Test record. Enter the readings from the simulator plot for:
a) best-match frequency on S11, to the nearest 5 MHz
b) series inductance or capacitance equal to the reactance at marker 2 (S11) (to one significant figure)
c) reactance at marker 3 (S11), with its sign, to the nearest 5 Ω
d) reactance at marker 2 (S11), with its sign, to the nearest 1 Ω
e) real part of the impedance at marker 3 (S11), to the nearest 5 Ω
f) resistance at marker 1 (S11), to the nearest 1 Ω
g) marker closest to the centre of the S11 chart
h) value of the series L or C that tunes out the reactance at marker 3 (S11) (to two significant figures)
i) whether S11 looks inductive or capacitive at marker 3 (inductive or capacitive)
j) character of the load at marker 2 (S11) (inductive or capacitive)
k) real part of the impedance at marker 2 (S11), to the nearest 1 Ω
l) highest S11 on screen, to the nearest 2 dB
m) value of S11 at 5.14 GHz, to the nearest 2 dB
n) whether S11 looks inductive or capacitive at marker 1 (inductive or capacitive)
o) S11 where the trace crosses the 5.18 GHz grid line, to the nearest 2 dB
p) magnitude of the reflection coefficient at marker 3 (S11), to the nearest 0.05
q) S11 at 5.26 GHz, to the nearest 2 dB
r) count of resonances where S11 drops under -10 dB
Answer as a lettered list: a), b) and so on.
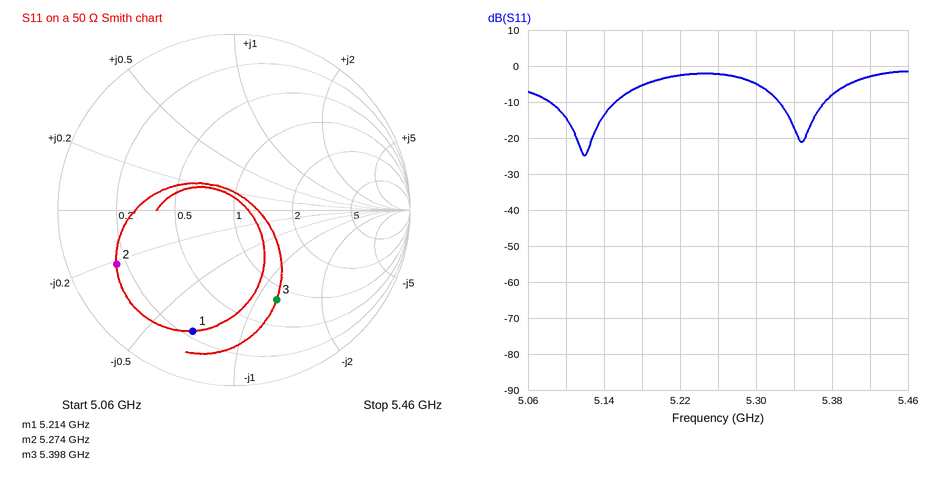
a) 5.120 GHz
b) 3 pF
c) -60 Ω
d) -11 Ω
e) 40 Ω
f) 12 Ω
g) marker 3
h) 1.8 nH
i) capacitive
j) capacitive
k) 8 Ω
l) -2 dB
m) -14 dB
n) capacitive
o) -6 dB
p) 0.55
q) -2 dB
r) 2
